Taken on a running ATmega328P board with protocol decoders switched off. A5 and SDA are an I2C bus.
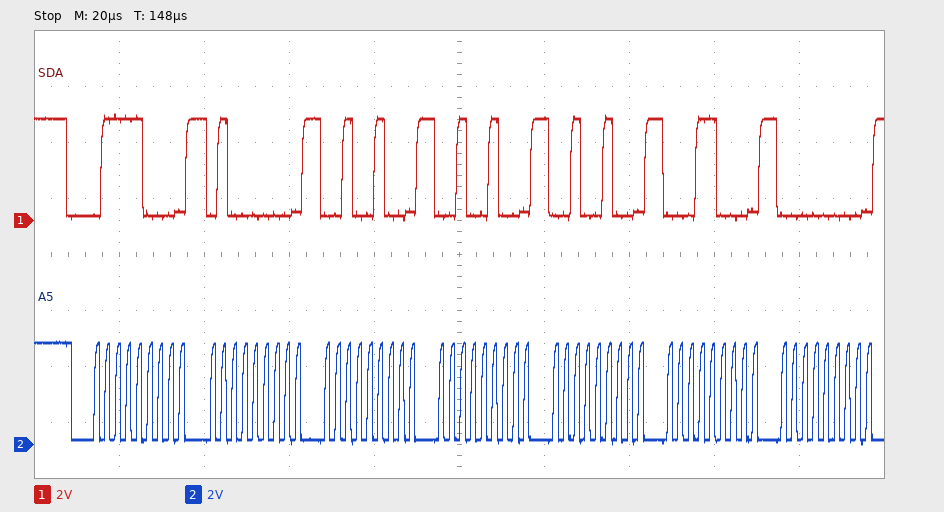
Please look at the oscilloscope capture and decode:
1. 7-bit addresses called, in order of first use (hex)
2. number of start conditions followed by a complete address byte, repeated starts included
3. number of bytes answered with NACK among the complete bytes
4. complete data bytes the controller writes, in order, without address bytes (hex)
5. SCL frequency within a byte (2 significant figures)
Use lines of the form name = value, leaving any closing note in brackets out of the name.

7-bit addresses called, in order of first use = 0x3C
number of start conditions followed by a complete address byte, repeated starts included = 1
number of bytes answered with NACK among the complete bytes = 0
complete data bytes the controller writes, in order, without address bytes = 40 24 24 24 18 00
SCL frequency within a byte = 400 kHz
